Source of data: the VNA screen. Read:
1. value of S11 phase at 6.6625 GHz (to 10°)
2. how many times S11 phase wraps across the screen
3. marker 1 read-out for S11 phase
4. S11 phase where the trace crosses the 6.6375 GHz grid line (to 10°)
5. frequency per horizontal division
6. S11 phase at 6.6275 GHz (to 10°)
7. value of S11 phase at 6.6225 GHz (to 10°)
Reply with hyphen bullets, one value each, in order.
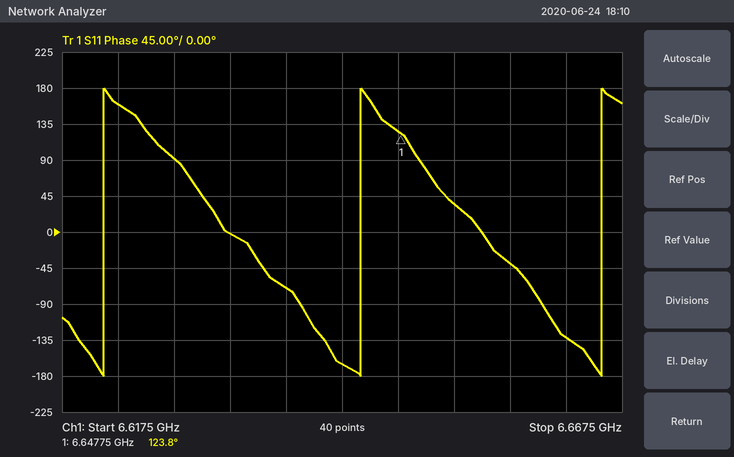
- -130°
- 3
- 123.8°
- -70°
- 5 MHz
- 90°
- 160°
